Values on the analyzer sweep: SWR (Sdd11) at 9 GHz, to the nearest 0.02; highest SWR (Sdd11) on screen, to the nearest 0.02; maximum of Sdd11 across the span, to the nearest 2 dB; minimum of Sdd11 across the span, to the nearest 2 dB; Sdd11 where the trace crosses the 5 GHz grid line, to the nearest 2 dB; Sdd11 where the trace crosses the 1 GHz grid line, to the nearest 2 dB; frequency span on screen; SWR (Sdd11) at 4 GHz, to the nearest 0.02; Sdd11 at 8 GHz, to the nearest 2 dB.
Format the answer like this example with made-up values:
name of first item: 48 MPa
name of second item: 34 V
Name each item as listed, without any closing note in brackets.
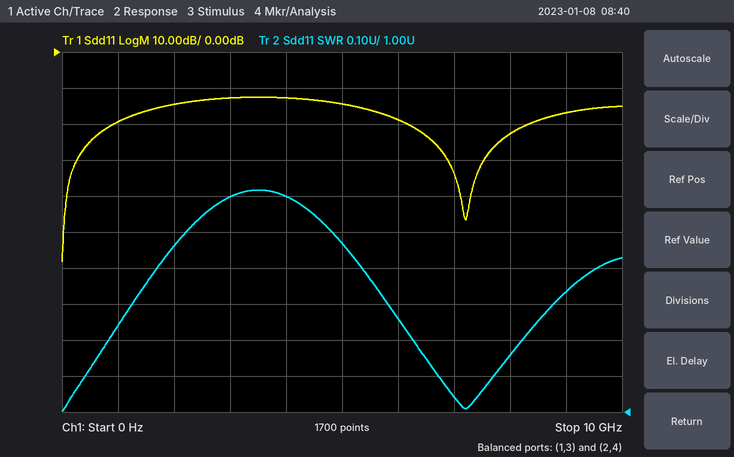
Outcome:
SWR (Sdd11) at 9 GHz, to the nearest 0.02: 1.34
highest SWR (Sdd11) on screen, to the nearest 0.02: 1.62
maximum of Sdd11 across the span, to the nearest 2 dB: -12 dB
minimum of Sdd11 across the span, to the nearest 2 dB: -58 dB
Sdd11 where the trace crosses the 5 GHz grid line, to the nearest 2 dB: -14 dB
Sdd11 where the trace crosses the 1 GHz grid line, to the nearest 2 dB: -20 dB
frequency span on screen: 10 GHz
SWR (Sdd11) at 4 GHz, to the nearest 0.02: 1.60
Sdd11 at 8 GHz, to the nearest 2 dB: -22 dB
